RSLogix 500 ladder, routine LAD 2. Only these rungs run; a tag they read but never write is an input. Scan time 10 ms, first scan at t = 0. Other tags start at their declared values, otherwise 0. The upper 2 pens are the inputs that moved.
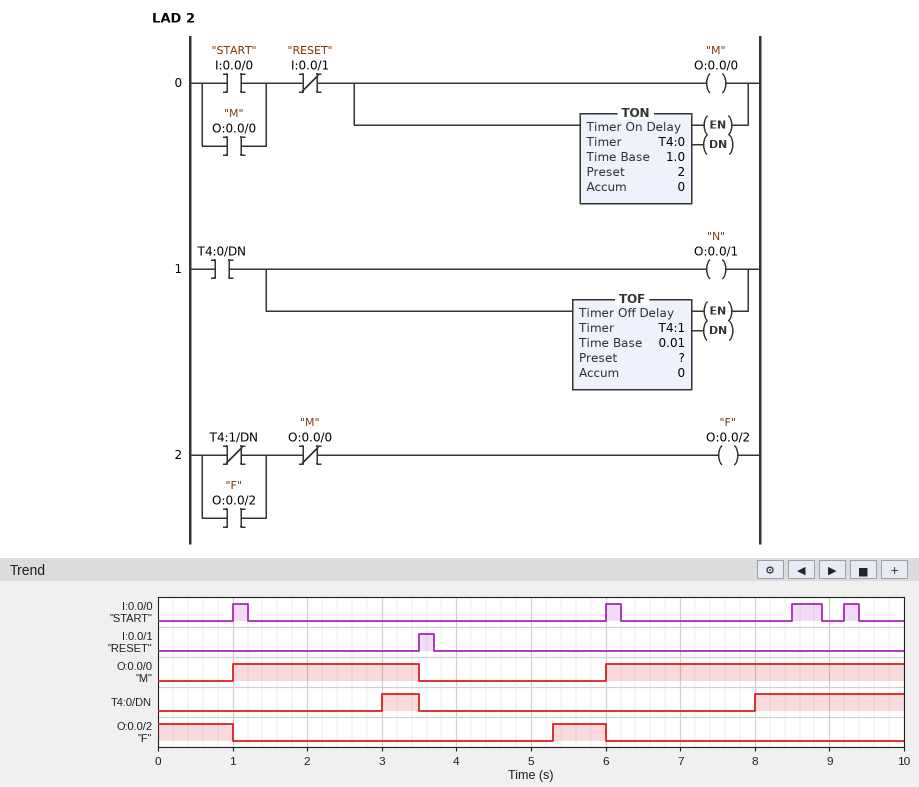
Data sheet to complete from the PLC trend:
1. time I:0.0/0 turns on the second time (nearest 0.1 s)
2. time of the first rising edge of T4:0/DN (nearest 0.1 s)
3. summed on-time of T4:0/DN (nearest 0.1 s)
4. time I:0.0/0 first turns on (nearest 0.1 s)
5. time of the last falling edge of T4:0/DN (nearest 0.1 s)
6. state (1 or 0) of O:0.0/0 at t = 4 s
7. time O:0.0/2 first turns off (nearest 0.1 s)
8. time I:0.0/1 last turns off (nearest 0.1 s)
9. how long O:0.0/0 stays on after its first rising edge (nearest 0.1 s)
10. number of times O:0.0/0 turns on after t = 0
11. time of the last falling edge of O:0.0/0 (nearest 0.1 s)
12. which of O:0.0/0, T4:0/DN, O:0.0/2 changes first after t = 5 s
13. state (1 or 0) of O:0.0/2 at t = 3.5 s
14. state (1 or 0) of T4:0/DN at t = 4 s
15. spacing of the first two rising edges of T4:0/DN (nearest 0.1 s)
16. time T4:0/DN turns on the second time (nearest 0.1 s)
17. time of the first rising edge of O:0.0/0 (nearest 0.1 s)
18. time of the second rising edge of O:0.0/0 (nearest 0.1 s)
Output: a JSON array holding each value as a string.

["6.0 s", "3.0 s", "2.5 s", "1.0 s", "3.5 s", "0", "1.0 s", "3.7 s", "2.5 s", "2", "3.5 s", "O:0.0/2", "0", "0", "5.0 s", "8.0 s", "1.0 s", "6.0 s"]
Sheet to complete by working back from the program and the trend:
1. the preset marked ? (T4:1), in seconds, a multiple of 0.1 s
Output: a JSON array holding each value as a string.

["1.8 s"]
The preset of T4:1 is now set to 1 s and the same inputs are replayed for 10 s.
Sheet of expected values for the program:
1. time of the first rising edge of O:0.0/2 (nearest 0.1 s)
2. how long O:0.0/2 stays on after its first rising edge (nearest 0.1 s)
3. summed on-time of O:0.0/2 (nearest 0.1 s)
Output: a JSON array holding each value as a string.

["4.5 s", "1.5 s", "2.5 s"]
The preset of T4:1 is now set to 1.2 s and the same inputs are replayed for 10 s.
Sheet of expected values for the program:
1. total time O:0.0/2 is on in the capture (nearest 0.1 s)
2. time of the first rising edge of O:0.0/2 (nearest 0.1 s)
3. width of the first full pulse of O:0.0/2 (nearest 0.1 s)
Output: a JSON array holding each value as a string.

["2.3 s", "4.7 s", "1.3 s"]
